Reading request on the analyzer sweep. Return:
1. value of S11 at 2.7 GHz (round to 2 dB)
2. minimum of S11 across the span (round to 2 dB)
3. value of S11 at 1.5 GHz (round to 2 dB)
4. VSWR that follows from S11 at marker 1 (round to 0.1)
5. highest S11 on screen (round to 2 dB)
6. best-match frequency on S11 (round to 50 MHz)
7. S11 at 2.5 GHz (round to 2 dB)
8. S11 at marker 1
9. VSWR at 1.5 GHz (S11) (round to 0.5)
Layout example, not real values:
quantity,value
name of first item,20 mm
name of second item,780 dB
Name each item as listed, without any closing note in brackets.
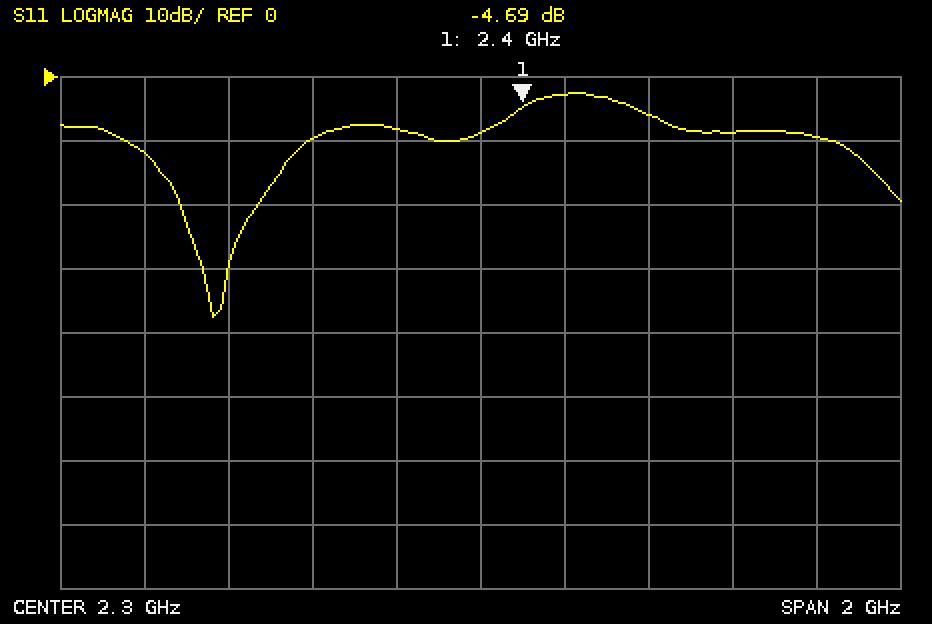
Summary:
quantity,value
value of S11 at 2.7 GHz,-6 dB
minimum of S11 across the span,-38 dB
value of S11 at 1.5 GHz,-12 dB
VSWR that follows from S11 at marker 1,3.8
highest S11 on screen,-2 dB
best-match frequency on S11,1.65 GHz
S11 at 2.5 GHz,-2 dB
S11 at marker 1,-4.69 dB
VSWR at 1.5 GHz (S11),1.5
